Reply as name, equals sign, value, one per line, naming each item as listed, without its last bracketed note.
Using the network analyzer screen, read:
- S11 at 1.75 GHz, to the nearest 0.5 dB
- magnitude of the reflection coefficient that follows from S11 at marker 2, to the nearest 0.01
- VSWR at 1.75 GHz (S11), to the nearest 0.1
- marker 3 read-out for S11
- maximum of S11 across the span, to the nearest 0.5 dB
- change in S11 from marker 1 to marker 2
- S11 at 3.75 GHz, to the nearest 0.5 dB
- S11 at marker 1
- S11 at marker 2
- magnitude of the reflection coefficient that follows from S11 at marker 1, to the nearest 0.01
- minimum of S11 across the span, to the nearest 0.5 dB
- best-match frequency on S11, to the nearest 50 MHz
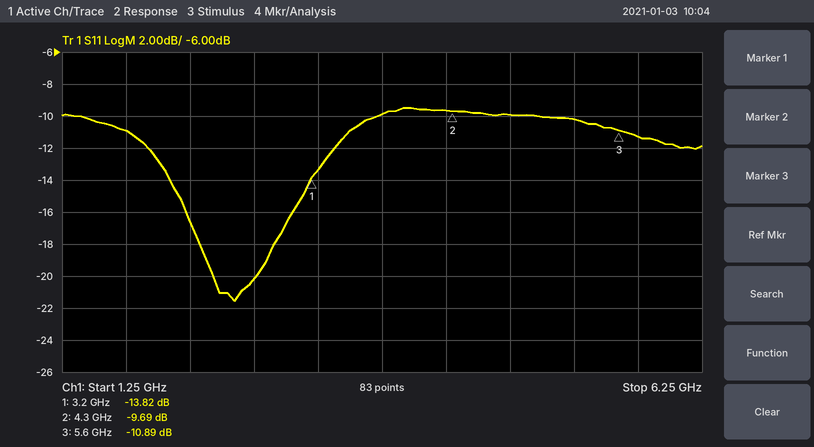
S11 at 1.75 GHz, to the nearest 0.5 dB = -11.0 dB
magnitude of the reflection coefficient that follows from S11 at marker 2, to the nearest 0.01 = 0.33
VSWR at 1.75 GHz (S11), to the nearest 0.1 = 1.8
marker 3 read-out for S11 = -10.89 dB
maximum of S11 across the span, to the nearest 0.5 dB = -9.5 dB
change in S11 from marker 1 to marker 2 = 4.13 dB
S11 at 3.75 GHz, to the nearest 0.5 dB = -10.0 dB
S11 at marker 1 = -13.82 dB
S11 at marker 2 = -9.69 dB
magnitude of the reflection coefficient that follows from S11 at marker 1, to the nearest 0.01 = 0.20
minimum of S11 across the span, to the nearest 0.5 dB = -21.5 dB
best-match frequency on S11, to the nearest 50 MHz = 2.60 GHz
